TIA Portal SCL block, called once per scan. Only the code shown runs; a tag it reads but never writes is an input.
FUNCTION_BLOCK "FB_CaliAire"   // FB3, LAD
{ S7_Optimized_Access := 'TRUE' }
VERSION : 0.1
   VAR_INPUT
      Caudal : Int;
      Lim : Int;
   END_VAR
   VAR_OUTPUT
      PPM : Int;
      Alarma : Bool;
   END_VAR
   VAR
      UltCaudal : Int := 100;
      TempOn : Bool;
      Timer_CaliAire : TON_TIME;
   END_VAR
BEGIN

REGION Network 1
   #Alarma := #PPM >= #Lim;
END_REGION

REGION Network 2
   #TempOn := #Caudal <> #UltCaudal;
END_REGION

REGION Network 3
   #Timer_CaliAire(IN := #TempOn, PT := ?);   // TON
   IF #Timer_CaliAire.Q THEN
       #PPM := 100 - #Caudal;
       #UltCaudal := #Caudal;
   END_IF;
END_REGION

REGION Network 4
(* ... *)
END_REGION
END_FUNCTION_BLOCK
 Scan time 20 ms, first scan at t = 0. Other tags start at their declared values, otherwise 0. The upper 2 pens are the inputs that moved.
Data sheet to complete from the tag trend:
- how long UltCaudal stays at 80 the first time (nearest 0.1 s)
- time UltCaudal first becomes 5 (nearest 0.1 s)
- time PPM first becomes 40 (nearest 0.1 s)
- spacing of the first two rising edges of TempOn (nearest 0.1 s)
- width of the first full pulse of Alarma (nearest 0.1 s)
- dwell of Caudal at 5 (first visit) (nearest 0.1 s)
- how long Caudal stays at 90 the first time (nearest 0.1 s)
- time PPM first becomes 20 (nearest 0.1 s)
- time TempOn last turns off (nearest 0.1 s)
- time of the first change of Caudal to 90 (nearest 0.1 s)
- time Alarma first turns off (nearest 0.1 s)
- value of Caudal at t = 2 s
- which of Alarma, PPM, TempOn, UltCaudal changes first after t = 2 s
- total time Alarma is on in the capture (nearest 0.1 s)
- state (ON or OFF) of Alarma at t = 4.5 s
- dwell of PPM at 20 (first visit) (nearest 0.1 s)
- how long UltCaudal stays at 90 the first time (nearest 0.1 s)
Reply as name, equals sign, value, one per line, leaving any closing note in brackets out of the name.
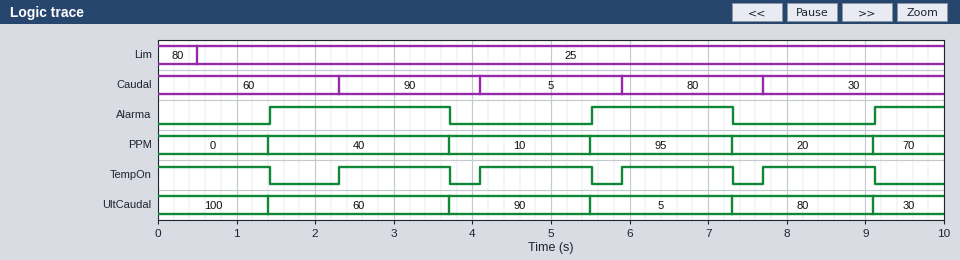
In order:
how long UltCaudal stays at 80 the first time = 1.8 s
time UltCaudal first becomes 5 = 5.5 s
time PPM first becomes 40 = 1.4 s
spacing of the first two rising edges of TempOn = 1.8 s
width of the first full pulse of Alarma = 2.3 s
dwell of Caudal at 5 (first visit) = 1.8 s
how long Caudal stays at 90 the first time = 1.8 s
time PPM first becomes 20 = 7.3 s
time TempOn last turns off = 9.1 s
time of the first change of Caudal to 90 = 2.3 s
time Alarma first turns off = 3.7 s
value of Caudal at t = 2 s = 60
which of Alarma, PPM, TempOn, UltCaudal changes first after t = 2 s = TempOn
total time Alarma is on in the capture = 5.0 s
state (ON or OFF) of Alarma at t = 4.5 s = OFF
dwell of PPM at 20 (first visit) = 1.8 s
how long UltCaudal stays at 90 the first time = 1.8 s
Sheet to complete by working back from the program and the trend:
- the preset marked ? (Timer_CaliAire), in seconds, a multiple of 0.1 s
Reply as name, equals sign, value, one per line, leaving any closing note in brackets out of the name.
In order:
the preset marked ? (Timer_CaliAire), in seconds, a multiple of 0.1 s = 1.4 s
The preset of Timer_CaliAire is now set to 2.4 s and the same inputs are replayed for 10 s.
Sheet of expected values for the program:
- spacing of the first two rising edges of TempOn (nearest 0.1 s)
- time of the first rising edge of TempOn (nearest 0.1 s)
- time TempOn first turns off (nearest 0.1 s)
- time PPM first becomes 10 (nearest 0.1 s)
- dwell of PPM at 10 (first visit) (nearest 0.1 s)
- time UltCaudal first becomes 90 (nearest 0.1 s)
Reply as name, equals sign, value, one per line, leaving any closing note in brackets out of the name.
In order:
spacing of the first two rising edges of TempOn = 3.6 s
time of the first rising edge of TempOn = 4.1 s
time TempOn first turns off = 2.4 s
time PPM first becomes 10 = 2.4 s
dwell of PPM at 10 (first visit) = 4.1 s
time UltCaudal first becomes 90 = 2.4 s
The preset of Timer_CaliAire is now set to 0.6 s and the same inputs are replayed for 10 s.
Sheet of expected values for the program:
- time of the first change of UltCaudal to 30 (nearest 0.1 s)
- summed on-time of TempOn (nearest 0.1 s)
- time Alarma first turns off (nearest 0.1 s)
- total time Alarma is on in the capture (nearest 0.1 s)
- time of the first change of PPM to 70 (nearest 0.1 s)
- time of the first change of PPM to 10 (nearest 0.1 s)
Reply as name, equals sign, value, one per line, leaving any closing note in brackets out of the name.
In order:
time of the first change of UltCaudal to 30 = 8.3 s
summed on-time of TempOn = 3.1 s
time Alarma first turns off = 2.9 s
total time Alarma is on in the capture = 5.8 s
time of the first change of PPM to 70 = 8.3 s
time of the first change of PPM to 10 = 2.9 s
